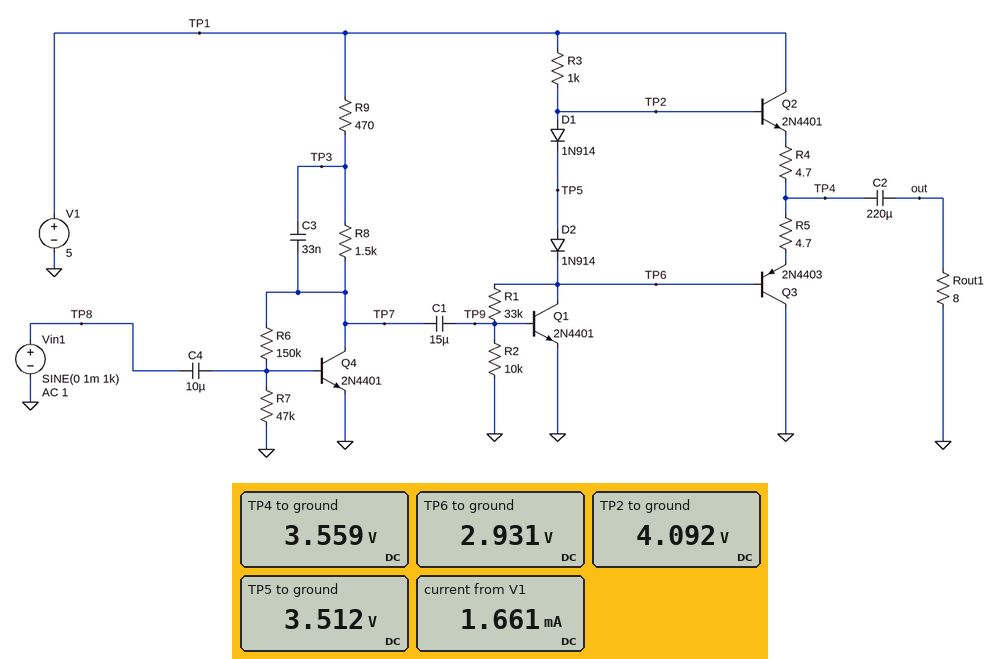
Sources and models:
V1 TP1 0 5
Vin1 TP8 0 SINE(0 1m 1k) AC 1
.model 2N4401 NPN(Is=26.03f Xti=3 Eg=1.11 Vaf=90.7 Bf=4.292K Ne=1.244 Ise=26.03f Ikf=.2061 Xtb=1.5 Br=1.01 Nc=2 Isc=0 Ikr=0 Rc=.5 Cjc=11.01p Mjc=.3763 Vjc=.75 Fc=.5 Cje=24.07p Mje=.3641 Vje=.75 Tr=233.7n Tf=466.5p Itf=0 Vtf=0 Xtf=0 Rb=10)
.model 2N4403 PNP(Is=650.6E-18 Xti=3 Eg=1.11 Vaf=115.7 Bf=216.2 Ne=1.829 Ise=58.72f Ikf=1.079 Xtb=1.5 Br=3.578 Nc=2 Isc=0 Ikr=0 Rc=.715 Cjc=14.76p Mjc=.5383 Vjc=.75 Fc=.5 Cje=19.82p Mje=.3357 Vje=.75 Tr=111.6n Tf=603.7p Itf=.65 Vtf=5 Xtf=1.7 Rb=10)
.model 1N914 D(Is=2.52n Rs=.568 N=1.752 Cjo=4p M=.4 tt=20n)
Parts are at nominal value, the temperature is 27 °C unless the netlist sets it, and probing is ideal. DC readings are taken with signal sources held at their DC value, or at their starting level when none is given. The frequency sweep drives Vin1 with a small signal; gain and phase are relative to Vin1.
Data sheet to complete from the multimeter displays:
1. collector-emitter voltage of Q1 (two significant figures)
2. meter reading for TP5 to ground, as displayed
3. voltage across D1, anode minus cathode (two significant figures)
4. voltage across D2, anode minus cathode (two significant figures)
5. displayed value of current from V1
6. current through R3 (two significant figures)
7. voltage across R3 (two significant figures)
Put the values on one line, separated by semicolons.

2.9 V; 3.512 V; 580 mV; 580 mV; 1.661 mA; 910 µA; 910 mV
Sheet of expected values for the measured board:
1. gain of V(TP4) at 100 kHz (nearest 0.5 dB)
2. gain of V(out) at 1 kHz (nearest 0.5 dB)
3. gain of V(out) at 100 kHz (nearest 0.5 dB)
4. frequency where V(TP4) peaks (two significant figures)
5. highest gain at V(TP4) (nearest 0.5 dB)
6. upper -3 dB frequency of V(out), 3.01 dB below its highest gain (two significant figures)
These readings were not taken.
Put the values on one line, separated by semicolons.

11.0 dB; 16.0 dB; 11.0 dB; 6.2 Hz; 36.0 dB; 11 kHz
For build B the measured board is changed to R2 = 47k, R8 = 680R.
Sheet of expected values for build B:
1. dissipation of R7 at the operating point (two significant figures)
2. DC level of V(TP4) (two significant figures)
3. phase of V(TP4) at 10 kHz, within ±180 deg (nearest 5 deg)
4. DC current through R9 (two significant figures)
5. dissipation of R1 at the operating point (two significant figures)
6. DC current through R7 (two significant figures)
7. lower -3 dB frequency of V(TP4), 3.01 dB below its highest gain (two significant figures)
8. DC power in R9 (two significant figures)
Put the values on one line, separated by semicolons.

8.4 µW; 2.3 V; -10 deg; 990 µA; 29 µW; 13 µA; 5.2 Hz; 460 µW
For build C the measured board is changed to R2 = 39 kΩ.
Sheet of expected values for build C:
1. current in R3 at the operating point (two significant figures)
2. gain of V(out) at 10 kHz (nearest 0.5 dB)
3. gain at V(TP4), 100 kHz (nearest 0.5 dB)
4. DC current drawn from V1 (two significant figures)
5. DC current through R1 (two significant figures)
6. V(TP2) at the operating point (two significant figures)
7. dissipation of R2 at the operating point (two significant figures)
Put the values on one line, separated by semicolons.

2.1 mA; 29.0 dB; 27.0 dB; 2.9 mA; 32 µA; 2.9 V; 11 µW
